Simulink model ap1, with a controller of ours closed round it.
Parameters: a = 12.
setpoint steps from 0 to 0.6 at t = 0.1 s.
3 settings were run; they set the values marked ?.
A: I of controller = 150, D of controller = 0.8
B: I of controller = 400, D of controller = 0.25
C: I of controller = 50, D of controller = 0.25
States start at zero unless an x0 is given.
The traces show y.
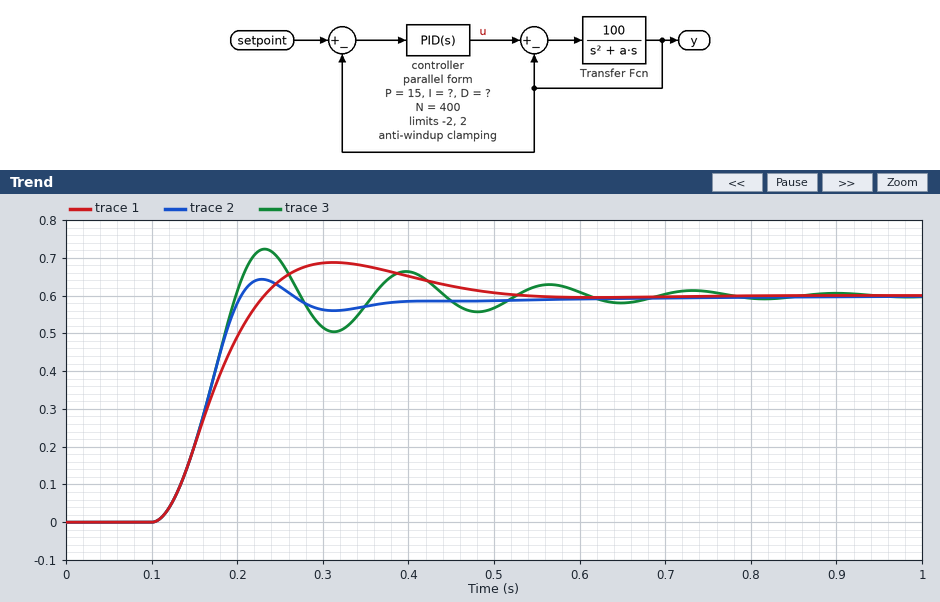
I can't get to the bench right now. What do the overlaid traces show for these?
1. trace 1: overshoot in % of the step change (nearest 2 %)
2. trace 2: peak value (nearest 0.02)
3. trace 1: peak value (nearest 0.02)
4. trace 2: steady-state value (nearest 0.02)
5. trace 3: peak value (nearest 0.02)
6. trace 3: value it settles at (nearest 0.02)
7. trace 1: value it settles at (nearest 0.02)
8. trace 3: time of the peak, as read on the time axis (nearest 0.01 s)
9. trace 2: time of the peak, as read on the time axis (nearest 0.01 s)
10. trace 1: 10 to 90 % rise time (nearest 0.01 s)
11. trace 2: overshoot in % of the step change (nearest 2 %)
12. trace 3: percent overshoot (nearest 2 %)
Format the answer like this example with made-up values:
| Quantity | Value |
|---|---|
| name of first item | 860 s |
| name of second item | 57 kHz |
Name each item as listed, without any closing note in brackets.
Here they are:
| Quantity | Value |
|---|---|
| trace 1: overshoot in % of the step change | 14 % |
| trace 2: peak value | 0.64 |
| trace 1: peak value | 0.68 |
| trace 2: steady-state value | 0.60 |
| trace 3: peak value | 0.72 |
| trace 3: value it settles at | 0.60 |
| trace 1: value it settles at | 0.60 |
| trace 3: time of the peak, as read on the time axis | 0.23 s |
| trace 2: time of the peak, as read on the time axis | 0.23 s |
| trace 1: 10 to 90 % rise time | 0.09 s |
| trace 2: overshoot in % of the step change | 8 % |
| trace 3: percent overshoot | 20 % |
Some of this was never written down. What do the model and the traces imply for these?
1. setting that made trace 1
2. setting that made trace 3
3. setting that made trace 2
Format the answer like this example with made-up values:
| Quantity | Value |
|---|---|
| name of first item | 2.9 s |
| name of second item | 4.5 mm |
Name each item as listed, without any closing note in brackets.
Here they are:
| Quantity | Value |
|---|---|
| setting that made trace 1 | A |
| setting that made trace 3 | B |
| setting that made trace 2 | C |
